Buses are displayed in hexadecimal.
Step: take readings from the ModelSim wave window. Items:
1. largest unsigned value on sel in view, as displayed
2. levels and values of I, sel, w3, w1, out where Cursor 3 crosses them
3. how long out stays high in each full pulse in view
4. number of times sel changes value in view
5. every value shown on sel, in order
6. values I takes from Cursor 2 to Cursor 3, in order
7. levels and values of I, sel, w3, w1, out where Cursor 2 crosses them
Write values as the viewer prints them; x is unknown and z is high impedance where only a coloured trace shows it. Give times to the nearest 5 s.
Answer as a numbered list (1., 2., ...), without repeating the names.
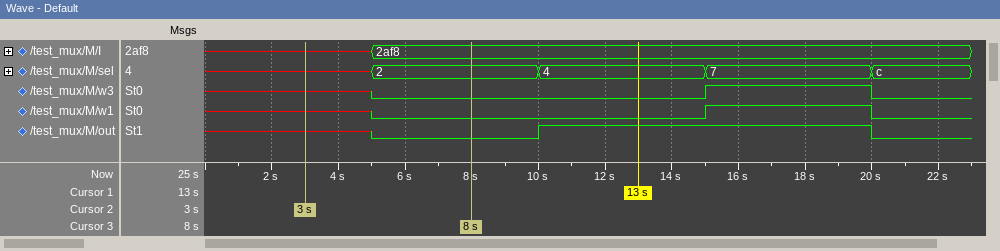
1. c
2. I=2af8, sel=2, w3=0, w1=0, out=0
3. 10 s
4. 4
5. x, 2, 4, 7, c
6. x, 2af8
7. I=x, sel=x, w3=x, w1=x, out=x
